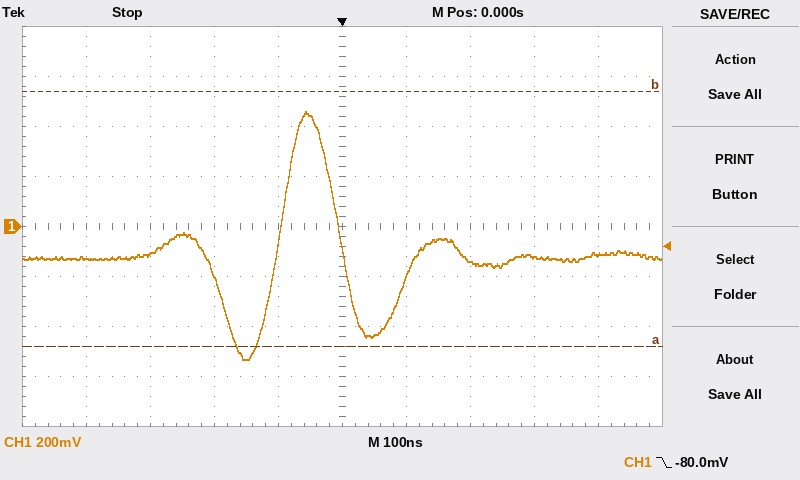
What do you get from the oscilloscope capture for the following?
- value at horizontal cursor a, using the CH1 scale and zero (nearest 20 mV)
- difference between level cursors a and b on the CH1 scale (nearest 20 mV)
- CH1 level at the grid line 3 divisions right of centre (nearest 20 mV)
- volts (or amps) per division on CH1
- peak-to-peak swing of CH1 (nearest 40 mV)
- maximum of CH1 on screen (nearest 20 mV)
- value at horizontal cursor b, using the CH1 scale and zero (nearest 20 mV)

-480 mV
1.02 V
-120 mV
200 mV
1.00 V
460 mV
540 mV
